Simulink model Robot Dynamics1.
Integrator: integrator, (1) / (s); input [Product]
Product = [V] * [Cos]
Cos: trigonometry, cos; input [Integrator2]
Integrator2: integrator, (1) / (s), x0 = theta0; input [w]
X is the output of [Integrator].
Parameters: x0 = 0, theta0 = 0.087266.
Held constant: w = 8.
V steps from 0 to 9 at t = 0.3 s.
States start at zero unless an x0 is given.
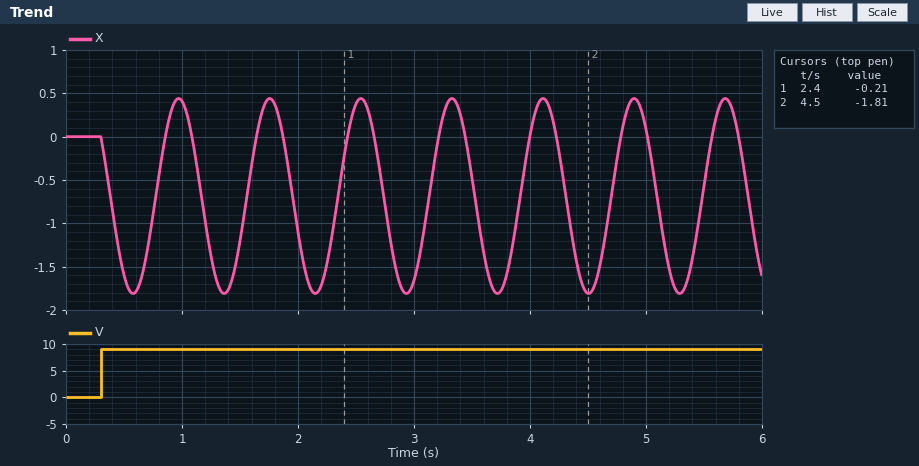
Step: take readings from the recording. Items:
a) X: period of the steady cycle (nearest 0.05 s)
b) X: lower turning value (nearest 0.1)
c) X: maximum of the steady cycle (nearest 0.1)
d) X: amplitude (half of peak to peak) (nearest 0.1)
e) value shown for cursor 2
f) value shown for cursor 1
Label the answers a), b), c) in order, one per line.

a) 0.80 s
b) -1.8
c) 0.4
d) 1.1
e) -1.81
f) -0.21
